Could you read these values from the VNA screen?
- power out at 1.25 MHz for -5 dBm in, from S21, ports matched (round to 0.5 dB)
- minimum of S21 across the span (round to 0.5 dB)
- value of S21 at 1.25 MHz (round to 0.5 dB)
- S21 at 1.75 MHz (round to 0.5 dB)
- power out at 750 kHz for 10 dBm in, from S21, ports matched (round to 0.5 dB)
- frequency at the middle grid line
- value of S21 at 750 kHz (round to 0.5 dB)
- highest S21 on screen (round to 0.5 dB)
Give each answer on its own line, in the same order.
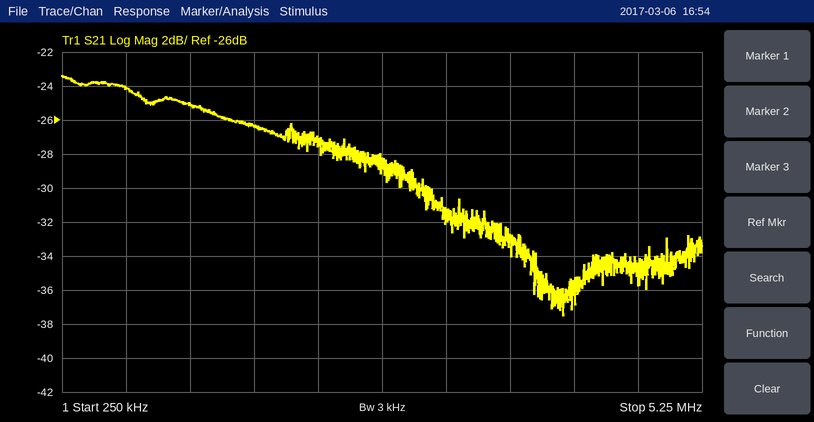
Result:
-30.0 dBm
-37.5 dB
-25.0 dB
-26.5 dB
-14.0 dBm
2.75 MHz
-24.0 dB
-23.5 dB
